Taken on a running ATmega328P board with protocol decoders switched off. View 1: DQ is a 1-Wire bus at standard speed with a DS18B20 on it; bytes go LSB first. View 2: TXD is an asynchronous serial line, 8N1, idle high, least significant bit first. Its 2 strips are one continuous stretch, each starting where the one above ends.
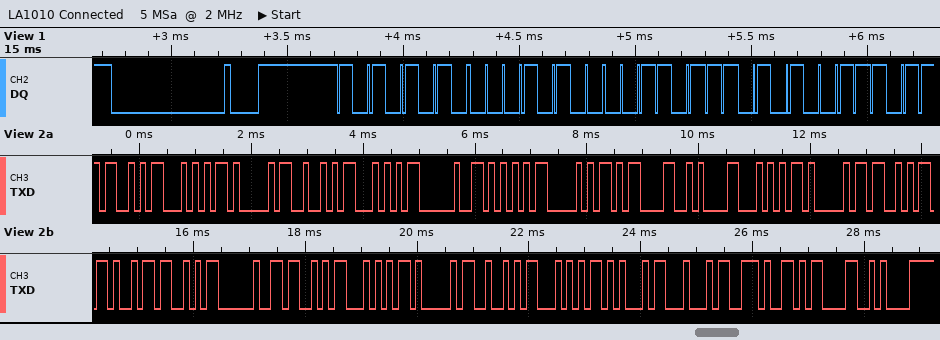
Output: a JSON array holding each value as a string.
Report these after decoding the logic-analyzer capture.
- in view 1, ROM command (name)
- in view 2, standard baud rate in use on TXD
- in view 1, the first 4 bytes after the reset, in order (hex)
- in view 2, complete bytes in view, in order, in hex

["Match ROM", "9600 baud", "55 28 EC CA", "53 54 41 52 54 20 55 50 0D 0A 54 41 53 4B 53 20 53 54 41 52 54 45 44 2E 0D 0A"]
